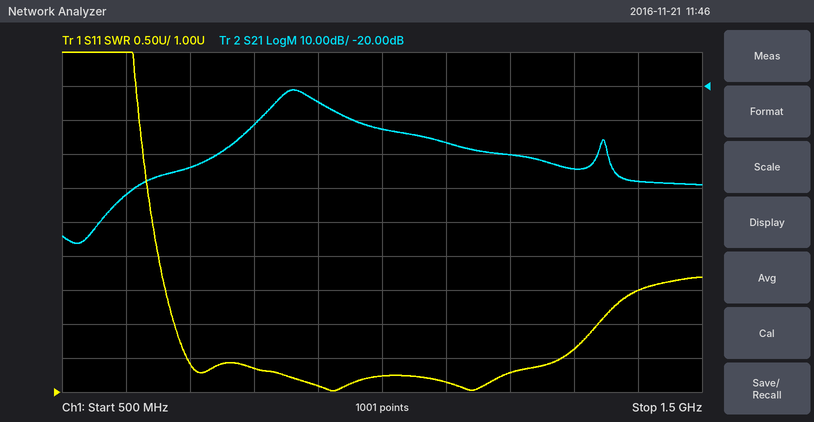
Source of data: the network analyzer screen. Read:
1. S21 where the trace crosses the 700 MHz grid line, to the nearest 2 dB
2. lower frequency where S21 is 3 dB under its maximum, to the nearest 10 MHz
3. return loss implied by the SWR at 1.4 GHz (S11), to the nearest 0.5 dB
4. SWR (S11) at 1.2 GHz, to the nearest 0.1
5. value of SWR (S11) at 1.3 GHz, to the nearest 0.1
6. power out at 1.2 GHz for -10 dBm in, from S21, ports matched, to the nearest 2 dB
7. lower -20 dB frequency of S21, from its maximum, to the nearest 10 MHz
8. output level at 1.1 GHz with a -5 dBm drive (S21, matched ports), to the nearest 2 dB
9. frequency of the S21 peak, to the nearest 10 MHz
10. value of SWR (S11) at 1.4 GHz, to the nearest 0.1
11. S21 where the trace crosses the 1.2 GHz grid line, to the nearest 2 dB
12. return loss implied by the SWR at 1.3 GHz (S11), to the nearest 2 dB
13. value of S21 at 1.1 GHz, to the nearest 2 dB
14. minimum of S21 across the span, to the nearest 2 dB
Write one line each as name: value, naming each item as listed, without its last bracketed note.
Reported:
S21 where the trace crosses the 700 MHz grid line, to the nearest 2 dB: -44 dB
lower frequency where S21 is 3 dB under its maximum, to the nearest 10 MHz: 840 MHz
return loss implied by the SWR at 1.4 GHz (S11), to the nearest 0.5 dB: 7.5 dB
SWR (S11) at 1.2 GHz, to the nearest 0.1: 1.3
value of SWR (S11) at 1.3 GHz, to the nearest 0.1: 1.6
power out at 1.2 GHz for -10 dBm in, from S21, ports matched, to the nearest 2 dB: -50 dBm
lower -20 dB frequency of S21, from its maximum, to the nearest 10 MHz: 730 MHz
output level at 1.1 GHz with a -5 dBm drive (S21, matched ports), to the nearest 2 dB: -42 dBm
frequency of the S21 peak, to the nearest 10 MHz: 860 MHz
value of SWR (S11) at 1.4 GHz, to the nearest 0.1: 2.5
S21 where the trace crosses the 1.2 GHz grid line, to the nearest 2 dB: -40 dB
return loss implied by the SWR at 1.3 GHz (S11), to the nearest 2 dB: 12 dB
value of S21 at 1.1 GHz, to the nearest 2 dB: -36 dB
minimum of S21 across the span, to the nearest 2 dB: -66 dB
